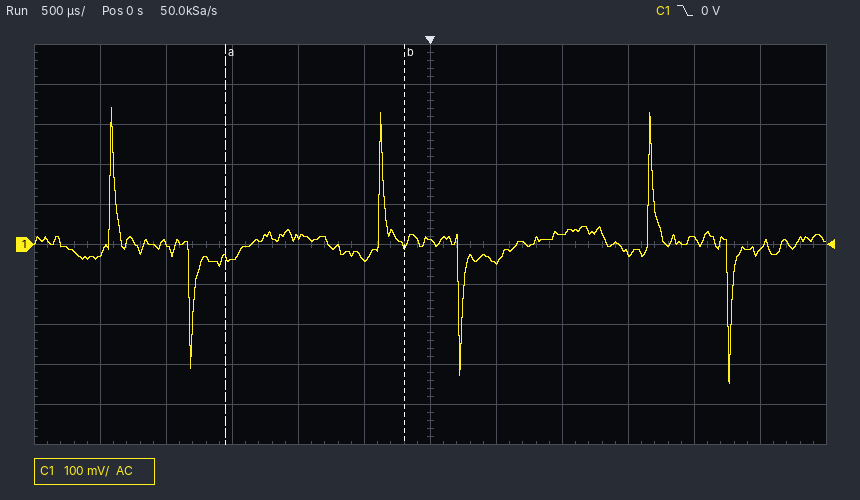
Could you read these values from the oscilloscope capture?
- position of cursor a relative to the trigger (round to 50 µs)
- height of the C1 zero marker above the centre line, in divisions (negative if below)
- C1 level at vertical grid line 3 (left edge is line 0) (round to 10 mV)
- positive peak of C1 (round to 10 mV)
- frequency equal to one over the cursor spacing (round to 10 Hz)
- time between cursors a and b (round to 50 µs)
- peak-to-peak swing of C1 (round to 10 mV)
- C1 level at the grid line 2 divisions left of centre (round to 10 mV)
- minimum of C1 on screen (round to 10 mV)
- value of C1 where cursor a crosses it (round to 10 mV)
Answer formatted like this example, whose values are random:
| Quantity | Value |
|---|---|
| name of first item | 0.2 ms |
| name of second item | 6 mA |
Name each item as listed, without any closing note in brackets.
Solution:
| Quantity | Value |
|---|---|
| position of cursor a relative to the trigger | -1.55 ms |
| height of the C1 zero marker above the centre line, in divisions | 0.0 div |
| C1 level at vertical grid line 3 (left edge is line 0) | -40 mV |
| positive peak of C1 | 340 mV |
| frequency equal to one over the cursor spacing | 740 Hz |
| time between cursors a and b | 1.35 ms |
| peak-to-peak swing of C1 | 690 mV |
| C1 level at the grid line 2 divisions left of centre | 20 mV |
| minimum of C1 on screen | -350 mV |
| value of C1 where cursor a crosses it | -30 mV |
